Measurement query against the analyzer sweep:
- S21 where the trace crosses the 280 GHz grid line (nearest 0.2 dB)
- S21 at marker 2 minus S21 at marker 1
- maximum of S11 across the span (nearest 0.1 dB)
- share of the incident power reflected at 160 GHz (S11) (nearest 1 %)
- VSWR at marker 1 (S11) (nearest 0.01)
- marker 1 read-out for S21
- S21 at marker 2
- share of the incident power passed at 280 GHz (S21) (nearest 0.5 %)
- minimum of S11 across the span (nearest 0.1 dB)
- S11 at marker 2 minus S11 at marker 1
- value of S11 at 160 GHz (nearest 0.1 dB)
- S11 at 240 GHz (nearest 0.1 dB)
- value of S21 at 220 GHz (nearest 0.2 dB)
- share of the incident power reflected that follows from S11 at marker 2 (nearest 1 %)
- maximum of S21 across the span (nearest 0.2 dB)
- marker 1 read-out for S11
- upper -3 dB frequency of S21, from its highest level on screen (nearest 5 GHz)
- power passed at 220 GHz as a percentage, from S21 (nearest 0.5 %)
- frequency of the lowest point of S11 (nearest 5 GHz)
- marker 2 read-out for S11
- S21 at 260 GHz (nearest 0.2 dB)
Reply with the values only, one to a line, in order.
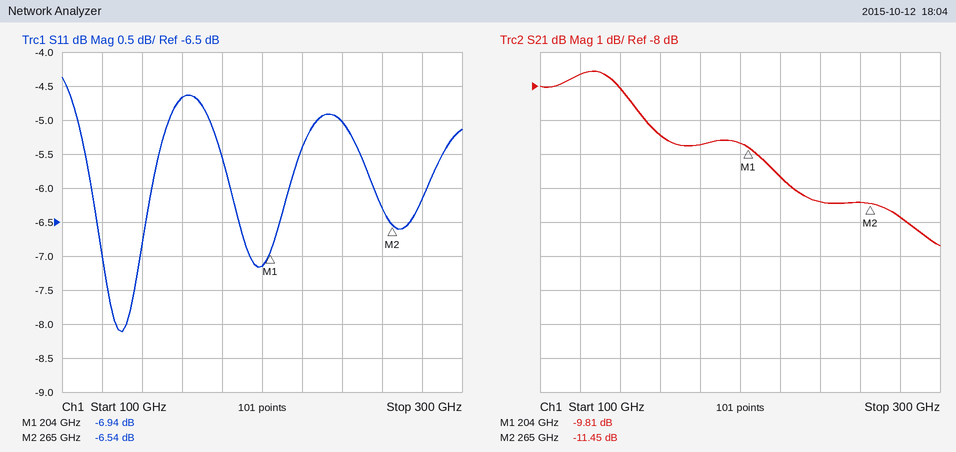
-11.8 dB
-1.64 dB
-4.4 dB
34 %
2.63
-9.81 dB
-11.45 dB
6.5 %
-8.1 dB
0.40 dB
-4.7 dB
-5.0 dB
-10.6 dB
22 %
-7.6 dB
-6.94 dB
220 GHz
8.5 %
130 GHz
-6.54 dB
-11.4 dB
